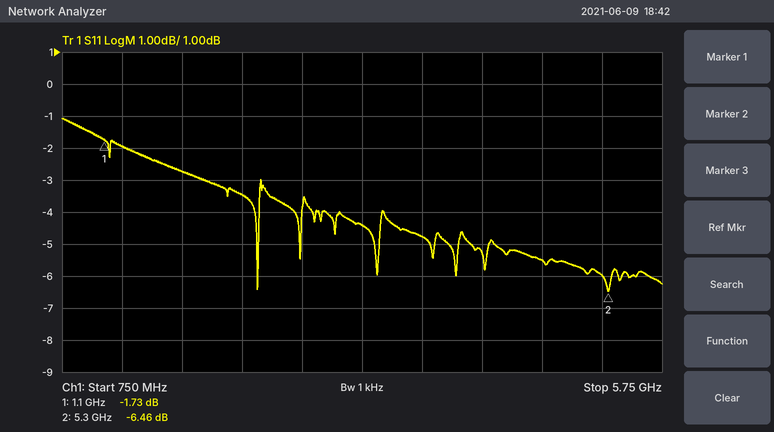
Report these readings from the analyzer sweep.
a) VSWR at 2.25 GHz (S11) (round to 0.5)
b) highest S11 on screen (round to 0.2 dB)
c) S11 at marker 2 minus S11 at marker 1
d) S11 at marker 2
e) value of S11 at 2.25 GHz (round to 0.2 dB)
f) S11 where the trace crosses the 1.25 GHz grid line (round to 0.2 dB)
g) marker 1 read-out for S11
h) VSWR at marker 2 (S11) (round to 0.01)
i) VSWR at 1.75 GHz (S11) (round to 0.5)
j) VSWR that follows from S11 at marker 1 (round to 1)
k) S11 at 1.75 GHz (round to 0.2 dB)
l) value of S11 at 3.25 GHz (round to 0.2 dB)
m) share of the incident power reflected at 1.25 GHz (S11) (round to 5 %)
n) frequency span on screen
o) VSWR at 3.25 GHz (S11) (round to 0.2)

5.0
-1.0 dB
-4.73 dB
-6.46 dB
-3.4 dB
-2.0 dB
-1.73 dB
2.81
6.5
10
-2.8 dB
-4.4 dB
65 %
5 GHz
4.0
